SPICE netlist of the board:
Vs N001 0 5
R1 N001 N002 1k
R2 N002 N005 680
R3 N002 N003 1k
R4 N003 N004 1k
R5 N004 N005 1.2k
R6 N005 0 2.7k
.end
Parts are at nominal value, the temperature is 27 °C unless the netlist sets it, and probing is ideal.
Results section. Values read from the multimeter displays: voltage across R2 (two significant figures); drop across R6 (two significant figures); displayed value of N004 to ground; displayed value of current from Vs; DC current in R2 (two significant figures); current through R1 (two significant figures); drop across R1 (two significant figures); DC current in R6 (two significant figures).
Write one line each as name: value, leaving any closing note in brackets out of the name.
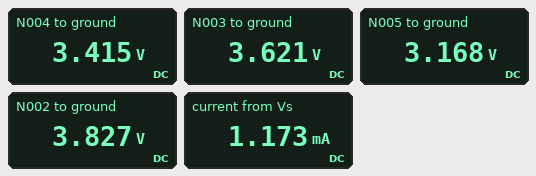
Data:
voltage across R2: 660 mV
drop across R6: 3.2 V
displayed value of N004 to ground: 3.415 V
displayed value of current from Vs: 1.173 mA
DC current in R2: 970 µA
current through R1: 1.2 mA
drop across R1: 1.2 V
DC current in R6: 1.2 mA
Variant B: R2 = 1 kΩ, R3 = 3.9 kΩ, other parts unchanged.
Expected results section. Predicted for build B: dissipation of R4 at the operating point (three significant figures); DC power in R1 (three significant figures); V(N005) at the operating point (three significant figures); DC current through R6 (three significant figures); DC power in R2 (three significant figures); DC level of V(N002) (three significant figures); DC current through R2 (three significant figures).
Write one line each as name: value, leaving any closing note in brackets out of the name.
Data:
dissipation of R4 at the operating point: 23.9 µW
DC power in R1: 1.20 mW
V(N005) at the operating point: 2.96 V
DC current through R6: 1.10 mA
DC power in R2: 888 µW
DC level of V(N002): 3.90 V
DC current through R2: 942 µA
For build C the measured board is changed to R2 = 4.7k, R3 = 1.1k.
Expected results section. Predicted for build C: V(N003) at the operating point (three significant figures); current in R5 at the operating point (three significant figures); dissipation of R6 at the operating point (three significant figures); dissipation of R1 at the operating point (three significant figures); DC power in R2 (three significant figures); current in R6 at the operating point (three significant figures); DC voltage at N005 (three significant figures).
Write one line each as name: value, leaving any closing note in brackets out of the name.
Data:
V(N003) at the operating point: 3.54 V
current in R5 at the operating point: 521 µA
dissipation of R6 at the operating point: 2.12 mW
dissipation of R1 at the operating point: 786 µW
DC power in R2: 629 µW
current in R6 at the operating point: 887 µA
DC voltage at N005: 2.39 V
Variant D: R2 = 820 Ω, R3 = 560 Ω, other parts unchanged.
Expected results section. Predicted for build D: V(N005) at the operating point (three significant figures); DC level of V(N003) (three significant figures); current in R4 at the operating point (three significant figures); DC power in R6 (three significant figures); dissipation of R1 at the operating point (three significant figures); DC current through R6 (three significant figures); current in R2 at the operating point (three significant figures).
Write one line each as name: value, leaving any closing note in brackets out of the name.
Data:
V(N005) at the operating point: 3.12 V
DC level of V(N003): 3.70 V
current in R4 at the operating point: 264 µA
DC power in R6: 3.60 mW
dissipation of R1 at the operating point: 1.33 mW
DC current through R6: 1.15 mA
current in R2 at the operating point: 890 µA
